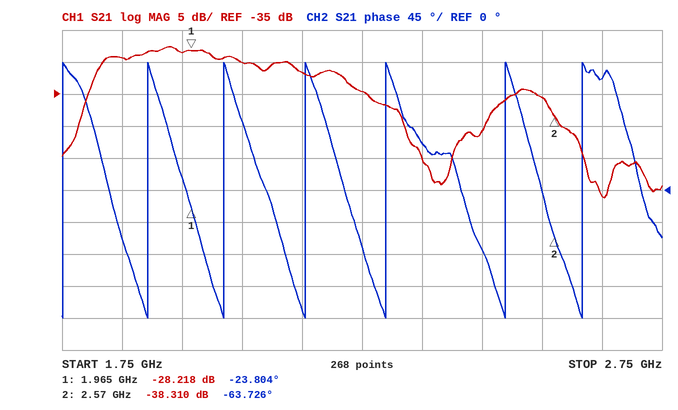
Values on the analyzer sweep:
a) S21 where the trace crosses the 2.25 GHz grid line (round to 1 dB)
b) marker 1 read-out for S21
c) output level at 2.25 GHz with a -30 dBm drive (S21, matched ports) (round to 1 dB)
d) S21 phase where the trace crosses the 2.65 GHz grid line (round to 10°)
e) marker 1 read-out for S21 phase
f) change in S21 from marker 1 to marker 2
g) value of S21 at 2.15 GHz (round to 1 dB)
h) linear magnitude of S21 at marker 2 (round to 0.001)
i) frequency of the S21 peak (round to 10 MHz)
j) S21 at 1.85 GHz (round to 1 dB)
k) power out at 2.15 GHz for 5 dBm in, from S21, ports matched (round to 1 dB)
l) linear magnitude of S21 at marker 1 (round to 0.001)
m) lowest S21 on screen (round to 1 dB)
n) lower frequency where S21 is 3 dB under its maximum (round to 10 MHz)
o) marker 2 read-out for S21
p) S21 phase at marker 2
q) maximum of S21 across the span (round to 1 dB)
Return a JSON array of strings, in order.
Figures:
["-35 dB", "-28.218 dB", "-65 dBm", "160°", "-23.804°", "-10.092 dB", "-32 dB", "0.012", "1.93 GHz", "-29 dB", "-27 dBm", "0.039", "-51 dB", "1.81 GHz", "-38.310 dB", "-63.726°", "-28 dB"]
